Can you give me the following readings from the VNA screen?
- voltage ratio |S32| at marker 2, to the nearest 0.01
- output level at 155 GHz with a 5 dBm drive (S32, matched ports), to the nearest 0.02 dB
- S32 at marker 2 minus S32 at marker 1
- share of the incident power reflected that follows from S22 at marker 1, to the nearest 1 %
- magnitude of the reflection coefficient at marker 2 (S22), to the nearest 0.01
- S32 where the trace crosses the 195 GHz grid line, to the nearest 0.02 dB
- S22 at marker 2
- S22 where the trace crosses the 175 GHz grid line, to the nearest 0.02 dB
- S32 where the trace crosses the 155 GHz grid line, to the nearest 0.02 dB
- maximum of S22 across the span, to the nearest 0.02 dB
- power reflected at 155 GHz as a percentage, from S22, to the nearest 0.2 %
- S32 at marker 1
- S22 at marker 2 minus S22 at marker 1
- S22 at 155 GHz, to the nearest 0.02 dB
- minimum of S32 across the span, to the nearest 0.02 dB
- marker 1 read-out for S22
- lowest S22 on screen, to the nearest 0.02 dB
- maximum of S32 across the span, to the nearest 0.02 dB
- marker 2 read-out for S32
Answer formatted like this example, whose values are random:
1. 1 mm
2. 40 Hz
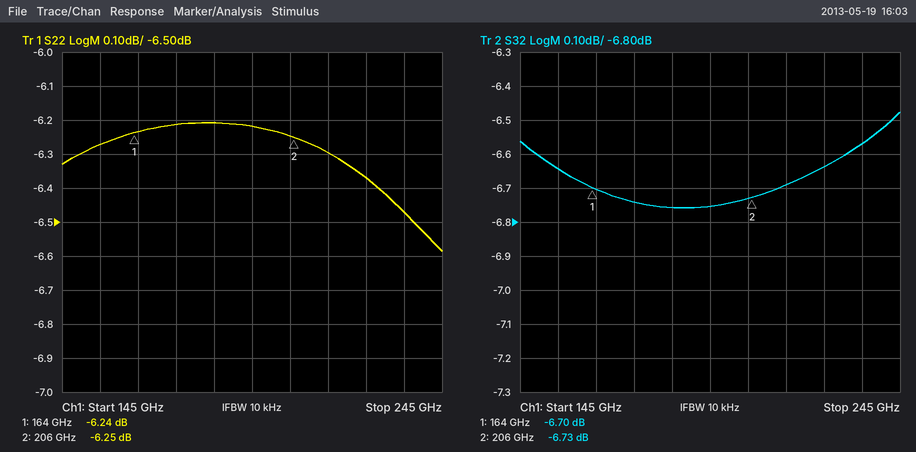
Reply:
1. 0.46
2. -1.64 dBm
3. -0.03 dB
4. 24 %
5. 0.49
6. -6.76 dB
7. -6.25 dB
8. -6.22 dB
9. -6.64 dB
10. -6.20 dB
11. 23.6 %
12. -6.70 dB
13. -0.01 dB
14. -6.28 dB
15. -6.76 dB
16. -6.24 dB
17. -6.58 dB
18. -6.48 dB
19. -6.73 dB
